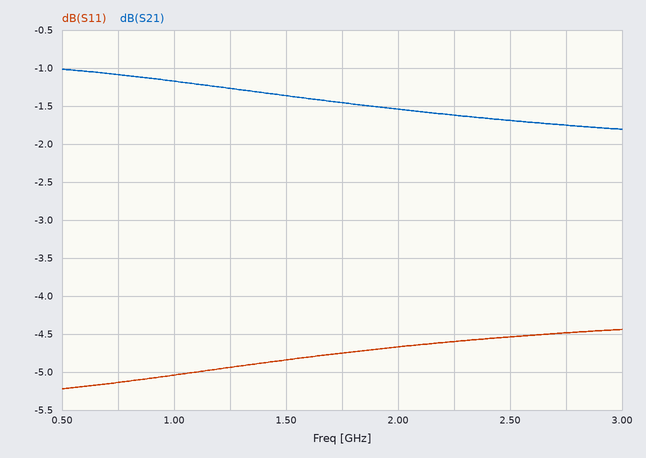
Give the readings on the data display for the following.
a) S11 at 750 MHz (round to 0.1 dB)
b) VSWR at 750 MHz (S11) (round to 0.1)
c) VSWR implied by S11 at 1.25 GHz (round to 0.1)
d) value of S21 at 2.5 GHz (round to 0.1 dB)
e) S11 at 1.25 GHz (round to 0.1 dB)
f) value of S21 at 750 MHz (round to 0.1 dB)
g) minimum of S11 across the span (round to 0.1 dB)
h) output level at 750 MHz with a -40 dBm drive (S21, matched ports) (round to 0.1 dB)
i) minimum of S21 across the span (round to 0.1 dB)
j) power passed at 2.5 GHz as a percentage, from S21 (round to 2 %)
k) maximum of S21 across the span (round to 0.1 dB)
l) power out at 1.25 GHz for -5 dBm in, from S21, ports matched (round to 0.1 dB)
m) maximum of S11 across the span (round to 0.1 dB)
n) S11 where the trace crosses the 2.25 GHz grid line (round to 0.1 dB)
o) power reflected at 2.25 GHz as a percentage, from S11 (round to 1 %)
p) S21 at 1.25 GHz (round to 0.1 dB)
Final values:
-5.1 dB
3.5
3.6
-1.7 dB
-4.9 dB
-1.1 dB
-5.2 dB
-41.1 dBm
-1.8 dB
68 %
-1.0 dB
-6.3 dBm
-4.4 dB
-4.6 dB
35 %
-1.3 dB
